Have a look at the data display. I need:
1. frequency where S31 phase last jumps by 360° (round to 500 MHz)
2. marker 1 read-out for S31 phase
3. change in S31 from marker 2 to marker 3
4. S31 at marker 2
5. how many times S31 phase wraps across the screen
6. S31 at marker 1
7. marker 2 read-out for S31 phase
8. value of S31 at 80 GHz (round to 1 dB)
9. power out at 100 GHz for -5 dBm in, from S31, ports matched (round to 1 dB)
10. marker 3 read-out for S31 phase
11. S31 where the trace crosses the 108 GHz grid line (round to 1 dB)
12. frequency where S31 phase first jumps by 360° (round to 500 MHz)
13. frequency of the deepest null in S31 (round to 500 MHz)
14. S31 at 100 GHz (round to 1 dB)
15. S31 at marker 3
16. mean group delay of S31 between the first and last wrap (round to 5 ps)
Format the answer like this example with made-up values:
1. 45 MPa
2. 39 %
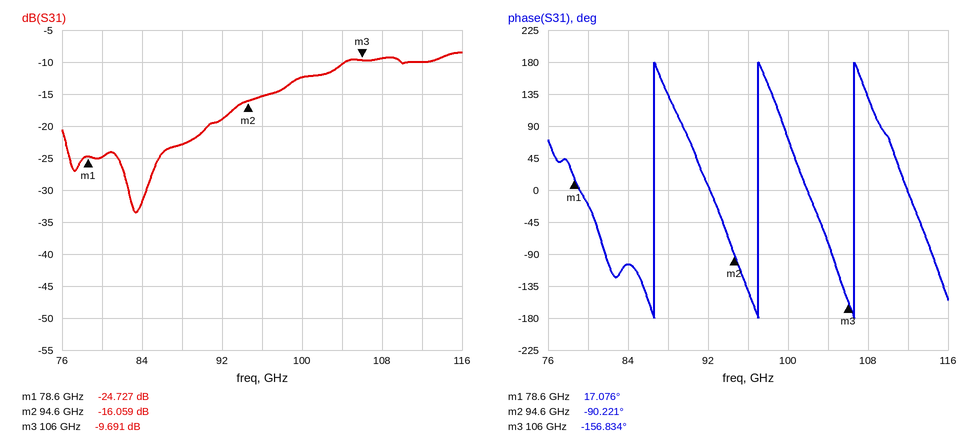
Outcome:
1. 106.5 GHz
2. 17.076°
3. 6.368 dB
4. -16.059 dB
5. 3
6. -24.727 dB
7. -90.221°
8. -25 dB
9. -17 dBm
10. -156.834°
11. -9 dB
12. 86.5 GHz
13. 83.5 GHz
14. -12 dB
15. -9.691 dB
16. 100 ps
